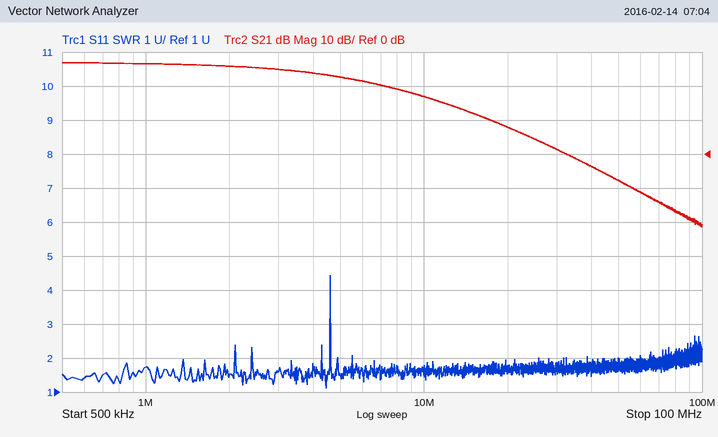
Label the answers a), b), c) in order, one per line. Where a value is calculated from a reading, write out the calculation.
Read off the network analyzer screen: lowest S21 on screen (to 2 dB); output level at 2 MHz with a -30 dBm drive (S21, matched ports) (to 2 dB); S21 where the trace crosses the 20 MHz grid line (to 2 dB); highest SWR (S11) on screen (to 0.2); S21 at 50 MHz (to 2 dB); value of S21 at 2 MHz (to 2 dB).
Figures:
a) -22 dB
b) -30 dBm + (26 dB) = -4 dBm
c) 8 dB
d) 4.4
e) -8 dB
f) 26 dB
